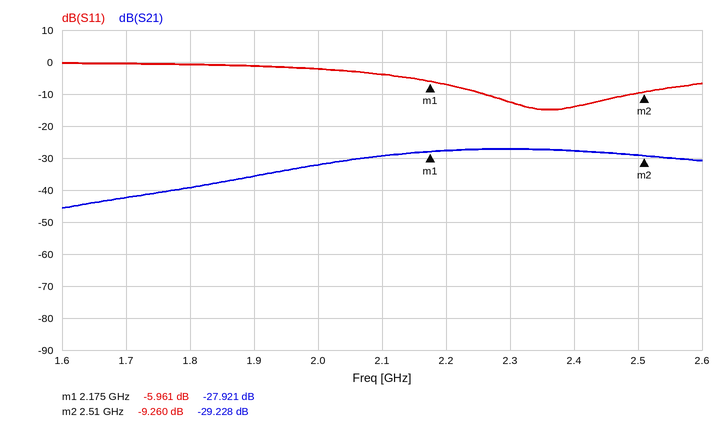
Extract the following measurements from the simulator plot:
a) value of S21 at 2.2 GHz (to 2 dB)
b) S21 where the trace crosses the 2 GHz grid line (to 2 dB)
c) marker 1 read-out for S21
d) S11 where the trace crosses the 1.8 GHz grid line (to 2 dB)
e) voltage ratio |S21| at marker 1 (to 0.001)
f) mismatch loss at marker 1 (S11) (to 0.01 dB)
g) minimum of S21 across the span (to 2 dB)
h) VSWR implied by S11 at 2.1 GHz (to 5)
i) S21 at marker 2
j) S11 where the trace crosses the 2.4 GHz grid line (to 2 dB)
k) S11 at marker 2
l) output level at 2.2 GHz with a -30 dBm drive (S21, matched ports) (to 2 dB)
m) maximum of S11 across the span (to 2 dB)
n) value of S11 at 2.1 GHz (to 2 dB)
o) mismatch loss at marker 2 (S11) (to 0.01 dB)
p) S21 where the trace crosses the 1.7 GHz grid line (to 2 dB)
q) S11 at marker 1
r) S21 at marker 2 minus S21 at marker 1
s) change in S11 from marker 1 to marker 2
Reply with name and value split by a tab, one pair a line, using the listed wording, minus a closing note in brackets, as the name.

value of S21 at 2.2 GHz	-28 dB
S21 where the trace crosses the 2 GHz grid line	-32 dB
marker 1 read-out for S21	-27.921 dB
S11 where the trace crosses the 1.8 GHz grid line	0 dB
voltage ratio |S21| at marker 1	0.040
mismatch loss at marker 1 (S11)	1.27 dB
minimum of S21 across the span	-46 dB
VSWR implied by S11 at 2.1 GHz	5
S21 at marker 2	-29.228 dB
S11 where the trace crosses the 2.4 GHz grid line	-14 dB
S11 at marker 2	-9.260 dB
output level at 2.2 GHz with a -30 dBm drive (S21, matched ports)	-58 dBm
maximum of S11 across the span	0 dB
value of S11 at 2.1 GHz	-4 dB
mismatch loss at marker 2 (S11)	0.55 dB
S21 where the trace crosses the 1.7 GHz grid line	-42 dB
S11 at marker 1	-5.961 dB
S21 at marker 2 minus S21 at marker 1	-1.307 dB
change in S11 from marker 1 to marker 2	-3.299 dB
